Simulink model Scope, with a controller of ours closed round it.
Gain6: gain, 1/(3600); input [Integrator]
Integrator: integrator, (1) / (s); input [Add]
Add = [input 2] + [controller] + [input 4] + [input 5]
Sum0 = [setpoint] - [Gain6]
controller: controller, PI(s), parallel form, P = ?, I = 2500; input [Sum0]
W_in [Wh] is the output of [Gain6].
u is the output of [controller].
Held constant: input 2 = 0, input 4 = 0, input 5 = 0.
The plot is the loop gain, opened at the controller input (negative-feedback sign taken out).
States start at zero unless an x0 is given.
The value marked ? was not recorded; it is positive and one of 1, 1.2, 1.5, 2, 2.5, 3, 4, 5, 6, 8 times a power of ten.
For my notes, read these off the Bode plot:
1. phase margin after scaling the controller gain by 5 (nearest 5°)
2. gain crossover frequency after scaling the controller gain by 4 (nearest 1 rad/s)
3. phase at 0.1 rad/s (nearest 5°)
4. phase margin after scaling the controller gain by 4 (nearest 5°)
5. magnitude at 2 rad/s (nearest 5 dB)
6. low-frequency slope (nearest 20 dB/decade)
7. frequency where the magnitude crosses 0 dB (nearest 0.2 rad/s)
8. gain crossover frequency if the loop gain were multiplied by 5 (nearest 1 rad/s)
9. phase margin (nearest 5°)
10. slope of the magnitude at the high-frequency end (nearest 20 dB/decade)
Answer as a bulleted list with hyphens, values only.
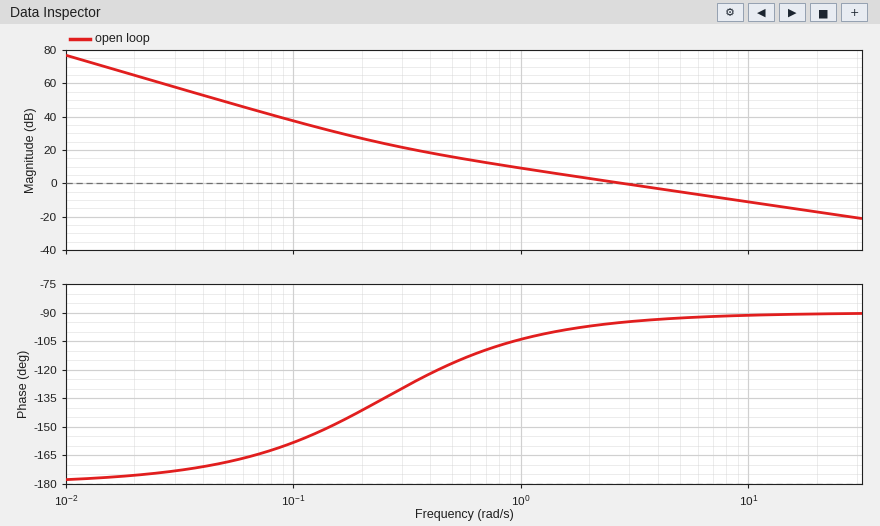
- 90°
- 11 rad/s
- -160°
- 90°
- 5 dB
- -40 dB/decade
- 2.8 rad/s
- 14 rad/s
- 85°
- -20 dB/decade
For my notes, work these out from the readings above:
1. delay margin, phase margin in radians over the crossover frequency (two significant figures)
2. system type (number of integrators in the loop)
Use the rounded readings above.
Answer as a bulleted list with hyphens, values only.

- 0.53 s
- 2
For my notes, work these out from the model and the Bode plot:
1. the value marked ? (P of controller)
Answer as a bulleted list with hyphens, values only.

- 10000
